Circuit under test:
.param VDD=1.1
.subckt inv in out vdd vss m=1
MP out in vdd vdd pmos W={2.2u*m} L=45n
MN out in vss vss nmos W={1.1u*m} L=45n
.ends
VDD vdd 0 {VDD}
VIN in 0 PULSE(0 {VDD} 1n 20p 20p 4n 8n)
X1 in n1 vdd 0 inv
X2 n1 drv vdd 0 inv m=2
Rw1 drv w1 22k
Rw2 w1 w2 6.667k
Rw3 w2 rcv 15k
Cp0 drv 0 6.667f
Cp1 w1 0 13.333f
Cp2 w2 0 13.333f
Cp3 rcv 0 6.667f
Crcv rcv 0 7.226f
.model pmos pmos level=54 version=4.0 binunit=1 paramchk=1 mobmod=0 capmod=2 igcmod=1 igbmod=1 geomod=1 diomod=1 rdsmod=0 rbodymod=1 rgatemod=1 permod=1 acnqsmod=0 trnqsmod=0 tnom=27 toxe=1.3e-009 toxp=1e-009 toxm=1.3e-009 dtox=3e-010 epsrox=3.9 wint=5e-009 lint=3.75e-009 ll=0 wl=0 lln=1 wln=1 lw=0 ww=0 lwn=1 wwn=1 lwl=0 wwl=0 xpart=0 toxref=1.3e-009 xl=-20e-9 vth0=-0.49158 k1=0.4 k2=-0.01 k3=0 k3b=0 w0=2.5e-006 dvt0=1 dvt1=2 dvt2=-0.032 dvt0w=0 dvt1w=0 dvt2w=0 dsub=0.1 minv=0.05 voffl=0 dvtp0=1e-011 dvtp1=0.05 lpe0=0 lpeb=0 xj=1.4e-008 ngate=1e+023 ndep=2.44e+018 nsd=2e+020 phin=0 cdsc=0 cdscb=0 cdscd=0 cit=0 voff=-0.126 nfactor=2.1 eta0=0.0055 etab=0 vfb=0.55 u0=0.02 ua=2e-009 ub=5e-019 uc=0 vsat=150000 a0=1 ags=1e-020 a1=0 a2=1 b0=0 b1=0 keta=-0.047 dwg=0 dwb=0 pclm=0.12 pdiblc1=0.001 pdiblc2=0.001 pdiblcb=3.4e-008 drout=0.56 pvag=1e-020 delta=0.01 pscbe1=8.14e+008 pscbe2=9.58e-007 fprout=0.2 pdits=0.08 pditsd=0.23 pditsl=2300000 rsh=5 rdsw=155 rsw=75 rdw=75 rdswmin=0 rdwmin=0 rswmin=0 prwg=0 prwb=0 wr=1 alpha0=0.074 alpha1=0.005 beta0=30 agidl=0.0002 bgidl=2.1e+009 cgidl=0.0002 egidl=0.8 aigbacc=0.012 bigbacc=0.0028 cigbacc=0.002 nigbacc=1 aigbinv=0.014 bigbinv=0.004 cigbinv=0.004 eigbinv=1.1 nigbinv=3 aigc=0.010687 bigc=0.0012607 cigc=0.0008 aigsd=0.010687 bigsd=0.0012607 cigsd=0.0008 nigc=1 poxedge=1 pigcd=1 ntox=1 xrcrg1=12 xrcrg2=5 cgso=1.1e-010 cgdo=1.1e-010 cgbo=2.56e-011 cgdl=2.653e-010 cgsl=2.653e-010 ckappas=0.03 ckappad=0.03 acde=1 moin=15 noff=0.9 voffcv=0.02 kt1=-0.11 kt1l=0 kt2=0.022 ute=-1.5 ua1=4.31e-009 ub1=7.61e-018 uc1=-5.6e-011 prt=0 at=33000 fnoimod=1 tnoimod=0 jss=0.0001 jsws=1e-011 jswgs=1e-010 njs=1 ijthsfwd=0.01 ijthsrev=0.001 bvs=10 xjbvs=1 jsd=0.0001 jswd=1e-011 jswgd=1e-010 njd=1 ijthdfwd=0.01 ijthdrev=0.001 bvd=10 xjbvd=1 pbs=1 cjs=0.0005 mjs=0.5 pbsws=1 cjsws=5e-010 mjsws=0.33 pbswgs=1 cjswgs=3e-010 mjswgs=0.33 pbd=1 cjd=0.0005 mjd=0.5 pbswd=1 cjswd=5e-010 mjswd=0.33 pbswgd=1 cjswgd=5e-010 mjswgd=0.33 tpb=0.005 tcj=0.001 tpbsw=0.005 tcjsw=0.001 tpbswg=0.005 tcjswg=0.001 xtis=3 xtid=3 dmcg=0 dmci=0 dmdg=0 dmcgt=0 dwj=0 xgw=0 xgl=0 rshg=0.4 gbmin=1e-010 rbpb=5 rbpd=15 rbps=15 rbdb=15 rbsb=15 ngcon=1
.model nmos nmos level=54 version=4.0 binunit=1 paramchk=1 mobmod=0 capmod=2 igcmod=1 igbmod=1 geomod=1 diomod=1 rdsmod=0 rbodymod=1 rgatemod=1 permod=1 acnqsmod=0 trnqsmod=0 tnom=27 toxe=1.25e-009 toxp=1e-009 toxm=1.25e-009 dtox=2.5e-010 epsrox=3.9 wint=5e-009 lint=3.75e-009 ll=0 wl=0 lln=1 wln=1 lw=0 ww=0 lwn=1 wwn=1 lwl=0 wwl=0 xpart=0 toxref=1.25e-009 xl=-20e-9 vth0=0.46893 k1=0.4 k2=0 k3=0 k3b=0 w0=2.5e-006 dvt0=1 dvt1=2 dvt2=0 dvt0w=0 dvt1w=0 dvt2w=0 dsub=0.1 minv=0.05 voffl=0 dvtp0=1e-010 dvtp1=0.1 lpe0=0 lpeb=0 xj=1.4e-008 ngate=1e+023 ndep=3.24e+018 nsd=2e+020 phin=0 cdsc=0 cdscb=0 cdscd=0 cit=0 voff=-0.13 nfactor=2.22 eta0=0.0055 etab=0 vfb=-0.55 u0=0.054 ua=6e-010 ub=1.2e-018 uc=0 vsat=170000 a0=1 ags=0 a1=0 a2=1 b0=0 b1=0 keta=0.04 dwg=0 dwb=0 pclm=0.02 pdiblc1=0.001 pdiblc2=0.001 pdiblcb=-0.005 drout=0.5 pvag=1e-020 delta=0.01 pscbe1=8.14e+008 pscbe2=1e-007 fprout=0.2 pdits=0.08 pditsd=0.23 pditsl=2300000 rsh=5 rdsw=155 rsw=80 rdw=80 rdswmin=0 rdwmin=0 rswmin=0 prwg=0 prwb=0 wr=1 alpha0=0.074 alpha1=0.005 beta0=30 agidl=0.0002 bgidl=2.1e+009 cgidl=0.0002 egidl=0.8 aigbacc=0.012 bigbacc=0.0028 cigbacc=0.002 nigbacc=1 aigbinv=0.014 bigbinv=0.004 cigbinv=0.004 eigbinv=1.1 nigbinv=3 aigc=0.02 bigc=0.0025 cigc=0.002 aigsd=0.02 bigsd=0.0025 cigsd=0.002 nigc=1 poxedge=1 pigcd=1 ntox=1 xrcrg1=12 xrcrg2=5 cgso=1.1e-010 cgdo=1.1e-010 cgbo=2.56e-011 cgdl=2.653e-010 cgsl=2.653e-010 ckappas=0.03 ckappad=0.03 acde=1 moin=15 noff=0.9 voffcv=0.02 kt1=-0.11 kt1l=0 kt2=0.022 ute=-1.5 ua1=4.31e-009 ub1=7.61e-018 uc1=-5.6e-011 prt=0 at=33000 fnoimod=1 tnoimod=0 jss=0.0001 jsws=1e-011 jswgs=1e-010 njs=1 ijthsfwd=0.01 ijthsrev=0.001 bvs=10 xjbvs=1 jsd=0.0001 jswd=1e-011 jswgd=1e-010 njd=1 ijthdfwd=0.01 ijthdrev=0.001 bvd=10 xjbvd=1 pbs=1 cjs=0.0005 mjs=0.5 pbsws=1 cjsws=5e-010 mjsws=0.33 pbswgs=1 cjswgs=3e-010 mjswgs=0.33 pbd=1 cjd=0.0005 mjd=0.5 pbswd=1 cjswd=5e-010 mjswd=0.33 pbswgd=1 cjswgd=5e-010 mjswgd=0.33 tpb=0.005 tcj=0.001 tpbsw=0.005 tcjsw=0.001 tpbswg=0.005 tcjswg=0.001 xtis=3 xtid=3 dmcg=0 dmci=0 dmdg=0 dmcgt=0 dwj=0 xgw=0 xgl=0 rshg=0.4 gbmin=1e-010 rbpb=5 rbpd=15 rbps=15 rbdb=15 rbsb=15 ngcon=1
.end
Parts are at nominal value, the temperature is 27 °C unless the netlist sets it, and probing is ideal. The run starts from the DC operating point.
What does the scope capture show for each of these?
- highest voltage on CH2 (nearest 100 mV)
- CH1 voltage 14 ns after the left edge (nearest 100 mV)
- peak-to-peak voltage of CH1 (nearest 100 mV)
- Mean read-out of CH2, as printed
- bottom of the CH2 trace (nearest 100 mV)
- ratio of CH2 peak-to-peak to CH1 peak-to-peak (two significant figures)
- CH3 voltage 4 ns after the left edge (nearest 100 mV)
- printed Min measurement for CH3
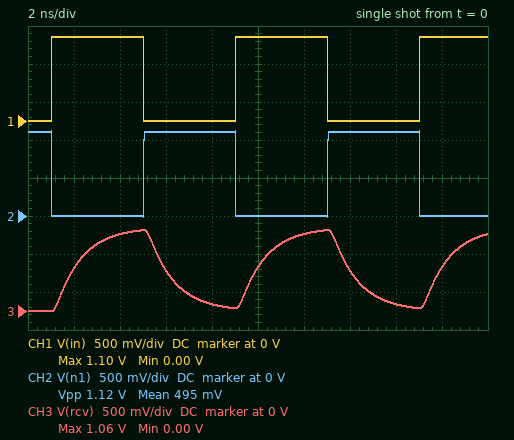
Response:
1.1 V
0 V
1.1 V
495 mV
0 V
1.0
1.0 V
0.00 V
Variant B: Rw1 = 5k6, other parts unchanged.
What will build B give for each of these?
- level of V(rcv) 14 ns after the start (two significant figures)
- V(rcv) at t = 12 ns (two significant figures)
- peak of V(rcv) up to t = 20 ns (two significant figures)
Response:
210 mV
1.1 V
1.1 V
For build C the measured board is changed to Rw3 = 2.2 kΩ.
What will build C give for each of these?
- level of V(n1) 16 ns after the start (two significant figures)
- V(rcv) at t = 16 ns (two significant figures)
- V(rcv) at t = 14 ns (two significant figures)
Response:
1.1 V
67 mV
460 mV
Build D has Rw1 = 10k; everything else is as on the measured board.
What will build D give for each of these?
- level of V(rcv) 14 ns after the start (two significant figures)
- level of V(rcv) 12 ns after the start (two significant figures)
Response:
320 mV
1.1 V
